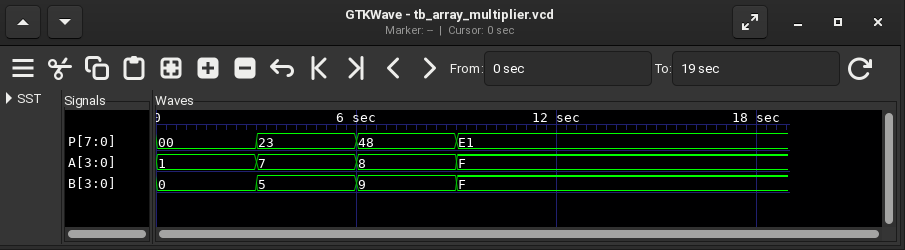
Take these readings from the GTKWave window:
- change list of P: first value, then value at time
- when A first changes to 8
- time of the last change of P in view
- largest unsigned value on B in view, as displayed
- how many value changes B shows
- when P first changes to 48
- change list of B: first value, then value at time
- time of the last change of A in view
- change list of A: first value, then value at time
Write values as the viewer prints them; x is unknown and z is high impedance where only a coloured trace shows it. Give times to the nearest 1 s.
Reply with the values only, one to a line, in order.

00, 23 at 3 s, 48 at 6 s, E1 at 9 s
6 s
9 s
F
3
6 s
0, 5 at 3 s, 9 at 6 s, F at 9 s
9 s
1, 7 at 3 s, 8 at 6 s, F at 9 s
